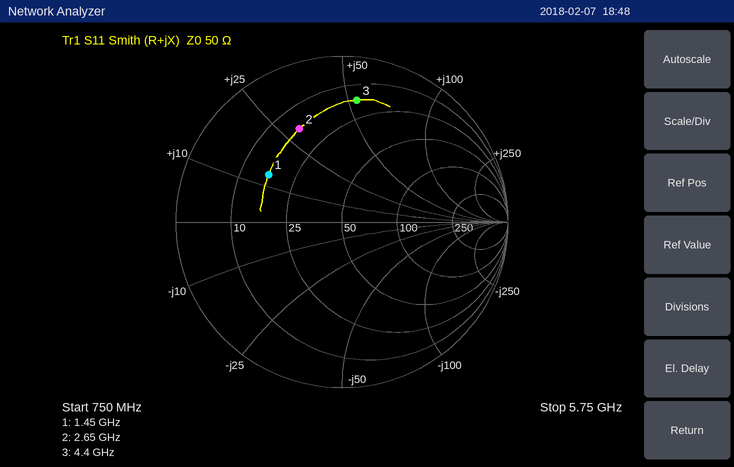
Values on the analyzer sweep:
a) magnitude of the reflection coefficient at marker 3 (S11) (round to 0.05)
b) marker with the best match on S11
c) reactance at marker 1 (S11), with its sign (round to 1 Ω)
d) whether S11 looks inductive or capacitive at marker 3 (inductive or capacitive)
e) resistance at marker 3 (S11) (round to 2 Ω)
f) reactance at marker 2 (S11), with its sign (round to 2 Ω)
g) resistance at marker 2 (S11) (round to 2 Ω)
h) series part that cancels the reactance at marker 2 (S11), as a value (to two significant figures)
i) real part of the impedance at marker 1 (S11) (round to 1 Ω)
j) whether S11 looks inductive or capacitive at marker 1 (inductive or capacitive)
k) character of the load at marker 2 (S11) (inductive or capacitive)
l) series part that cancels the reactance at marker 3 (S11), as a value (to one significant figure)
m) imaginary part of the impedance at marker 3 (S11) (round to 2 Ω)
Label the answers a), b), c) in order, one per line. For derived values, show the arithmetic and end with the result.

a) 0.75
b) marker 1
c) +13 Ω
d) inductive
e) 16 Ω
f) +30 Ω
g) 16 Ω
h) C = 1/(2π × 2.65 GHz × 30 Ω) ≈ 2.0 pF
i) 17 Ω
j) inductive
k) inductive
l) C = 1/(2π × 4.4 GHz × 54 Ω) ≈ 670 fF, so 700 fF to one significant figure
m) +54 Ω
